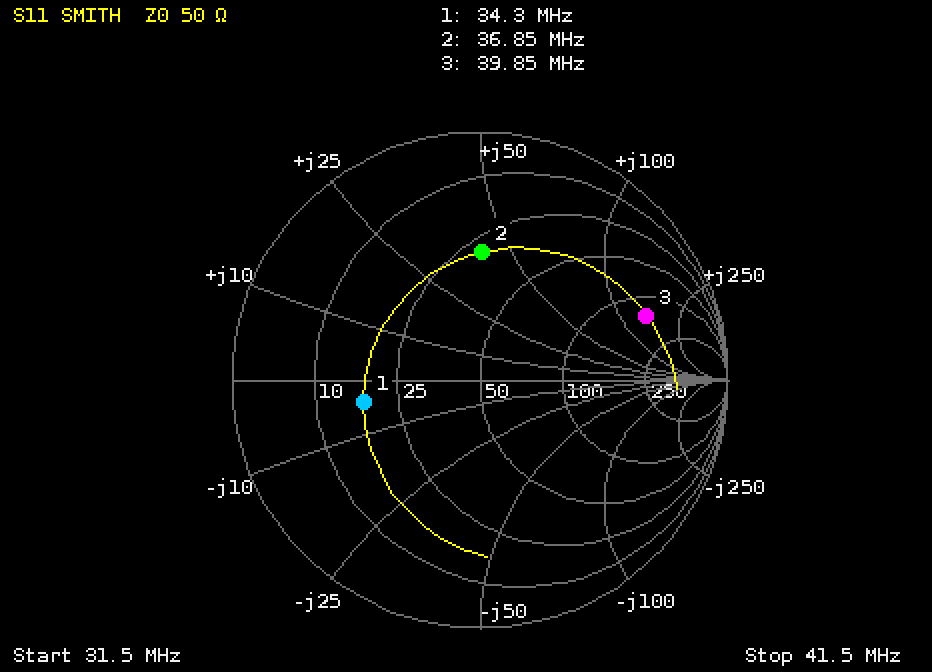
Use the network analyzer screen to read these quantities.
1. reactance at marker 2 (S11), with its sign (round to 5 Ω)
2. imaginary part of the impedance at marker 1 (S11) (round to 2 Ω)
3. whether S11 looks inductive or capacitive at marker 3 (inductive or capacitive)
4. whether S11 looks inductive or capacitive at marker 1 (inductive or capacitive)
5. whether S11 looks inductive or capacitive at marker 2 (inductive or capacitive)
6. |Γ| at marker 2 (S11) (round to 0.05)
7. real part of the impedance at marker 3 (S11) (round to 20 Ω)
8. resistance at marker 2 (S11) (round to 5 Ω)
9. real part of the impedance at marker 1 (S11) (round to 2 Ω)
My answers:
+40 Ω
-4 Ω
inductive
capacitive
inductive
0.50
140 Ω
30 Ω
18 Ω
